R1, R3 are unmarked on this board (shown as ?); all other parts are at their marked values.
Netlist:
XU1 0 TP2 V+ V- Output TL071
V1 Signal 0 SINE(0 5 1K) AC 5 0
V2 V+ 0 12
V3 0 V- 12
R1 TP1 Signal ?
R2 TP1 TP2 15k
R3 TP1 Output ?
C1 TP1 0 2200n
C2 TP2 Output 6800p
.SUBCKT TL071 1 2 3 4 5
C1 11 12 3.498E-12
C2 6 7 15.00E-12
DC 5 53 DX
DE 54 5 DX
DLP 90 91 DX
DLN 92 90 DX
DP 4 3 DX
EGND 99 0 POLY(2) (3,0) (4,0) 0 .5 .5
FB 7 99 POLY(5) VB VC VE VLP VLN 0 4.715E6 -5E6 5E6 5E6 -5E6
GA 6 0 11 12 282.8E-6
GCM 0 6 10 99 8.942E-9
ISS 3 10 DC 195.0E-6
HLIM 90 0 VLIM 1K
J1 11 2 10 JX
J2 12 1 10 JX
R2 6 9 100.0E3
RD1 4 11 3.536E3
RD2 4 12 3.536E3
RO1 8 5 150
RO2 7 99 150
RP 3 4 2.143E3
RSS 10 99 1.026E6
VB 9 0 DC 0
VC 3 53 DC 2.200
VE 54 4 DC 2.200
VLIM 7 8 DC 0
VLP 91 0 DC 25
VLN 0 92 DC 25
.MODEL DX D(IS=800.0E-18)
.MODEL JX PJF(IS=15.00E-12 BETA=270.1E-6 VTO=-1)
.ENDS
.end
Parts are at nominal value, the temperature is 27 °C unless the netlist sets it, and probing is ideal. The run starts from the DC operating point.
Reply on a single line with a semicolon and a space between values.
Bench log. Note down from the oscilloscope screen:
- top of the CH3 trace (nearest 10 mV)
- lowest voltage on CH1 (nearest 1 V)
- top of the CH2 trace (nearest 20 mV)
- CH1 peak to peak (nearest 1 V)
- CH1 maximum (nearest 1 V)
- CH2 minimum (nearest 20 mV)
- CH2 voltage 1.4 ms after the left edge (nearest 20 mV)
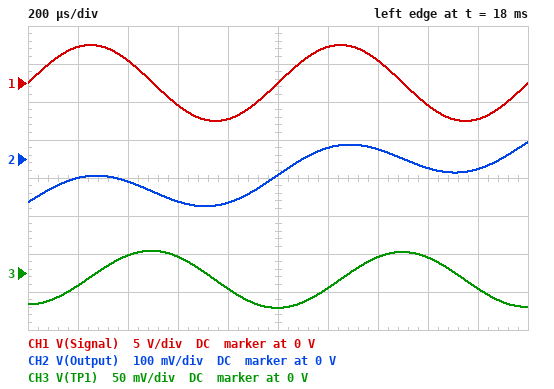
30 mV; -5 V; 40 mV; 10 V; 5 V; -120 mV; 20 mV
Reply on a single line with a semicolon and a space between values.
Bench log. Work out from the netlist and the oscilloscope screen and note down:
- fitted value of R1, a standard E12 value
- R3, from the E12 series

10 kΩ; 6.8 kΩ
